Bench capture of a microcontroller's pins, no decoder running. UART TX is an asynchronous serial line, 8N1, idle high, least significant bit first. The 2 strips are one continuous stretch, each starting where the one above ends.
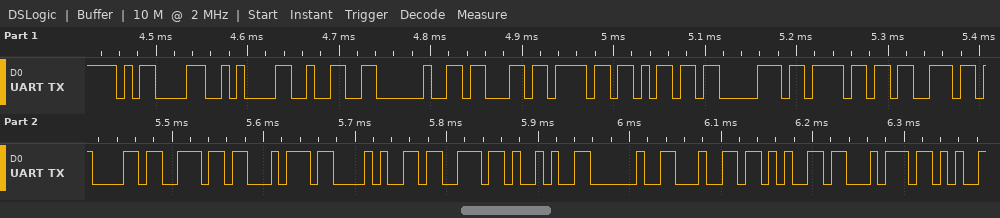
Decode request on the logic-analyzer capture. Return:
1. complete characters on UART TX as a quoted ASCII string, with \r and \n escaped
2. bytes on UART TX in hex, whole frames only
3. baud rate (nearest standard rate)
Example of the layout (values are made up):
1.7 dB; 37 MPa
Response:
"\r\n2 composant(s) det"; 0D 0A 32 20 63 6F 6D 70 6F 73 61 6E 74 28 73 29 20 64 65 74; 115200 baud
